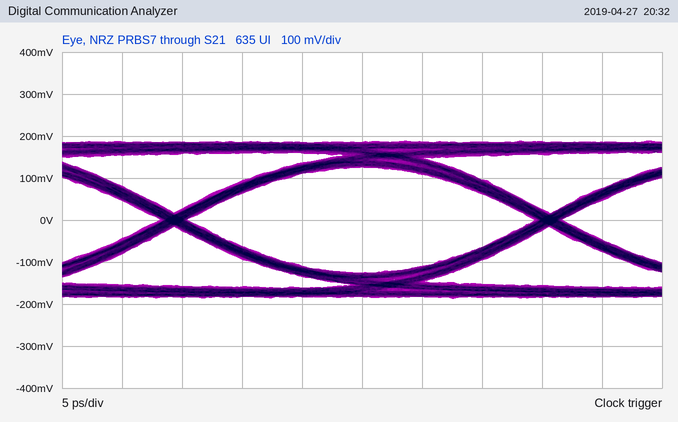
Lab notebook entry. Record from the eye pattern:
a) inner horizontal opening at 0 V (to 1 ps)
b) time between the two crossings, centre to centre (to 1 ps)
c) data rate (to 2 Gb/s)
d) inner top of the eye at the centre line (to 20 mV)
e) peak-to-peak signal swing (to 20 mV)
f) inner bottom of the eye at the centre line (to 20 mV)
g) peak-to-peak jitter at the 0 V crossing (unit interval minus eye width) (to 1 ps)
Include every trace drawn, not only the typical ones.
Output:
29 ps
31 ps
32 Gb/s
120 mV
380 mV
-120 mV
2 ps
